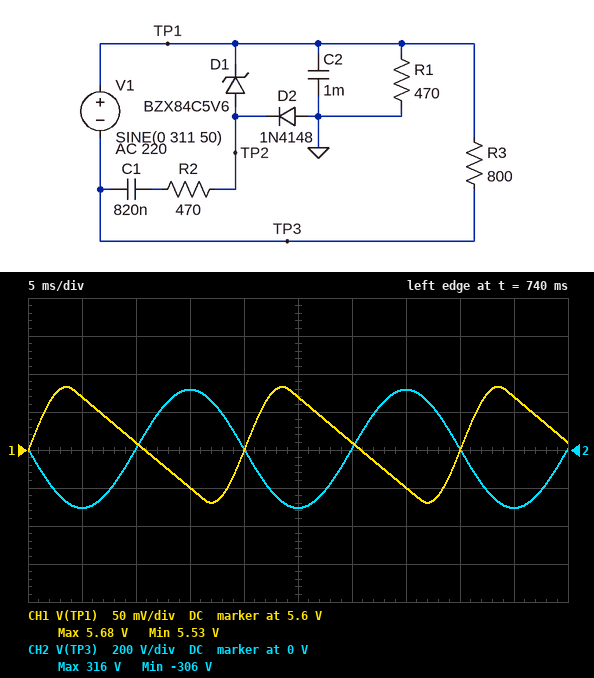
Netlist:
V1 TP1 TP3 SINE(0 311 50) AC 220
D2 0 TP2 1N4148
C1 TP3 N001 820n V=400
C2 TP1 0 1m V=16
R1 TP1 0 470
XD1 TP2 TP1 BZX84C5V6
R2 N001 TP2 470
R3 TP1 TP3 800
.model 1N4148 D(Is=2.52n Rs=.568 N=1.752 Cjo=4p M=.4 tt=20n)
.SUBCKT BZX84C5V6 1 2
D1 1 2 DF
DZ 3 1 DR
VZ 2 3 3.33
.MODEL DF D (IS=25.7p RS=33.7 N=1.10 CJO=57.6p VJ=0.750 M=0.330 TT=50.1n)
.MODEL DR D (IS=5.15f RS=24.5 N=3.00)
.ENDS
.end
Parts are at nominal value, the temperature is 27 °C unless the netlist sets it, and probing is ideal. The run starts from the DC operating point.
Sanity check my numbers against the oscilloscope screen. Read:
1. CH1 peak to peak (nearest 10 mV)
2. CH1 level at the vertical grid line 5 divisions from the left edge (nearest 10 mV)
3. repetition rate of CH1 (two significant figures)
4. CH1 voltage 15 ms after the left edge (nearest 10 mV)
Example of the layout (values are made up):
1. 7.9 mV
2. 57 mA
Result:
1. 150 mV
2. 5.67 V
3. 50 Hz
4. 5.55 V
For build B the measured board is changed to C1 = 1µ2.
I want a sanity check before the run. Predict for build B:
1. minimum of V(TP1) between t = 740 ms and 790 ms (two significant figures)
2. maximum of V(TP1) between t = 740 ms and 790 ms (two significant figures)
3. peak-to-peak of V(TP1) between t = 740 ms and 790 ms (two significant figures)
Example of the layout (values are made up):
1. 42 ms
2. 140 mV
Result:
1. 6.2 V
2. 6.3 V
3. 180 mV
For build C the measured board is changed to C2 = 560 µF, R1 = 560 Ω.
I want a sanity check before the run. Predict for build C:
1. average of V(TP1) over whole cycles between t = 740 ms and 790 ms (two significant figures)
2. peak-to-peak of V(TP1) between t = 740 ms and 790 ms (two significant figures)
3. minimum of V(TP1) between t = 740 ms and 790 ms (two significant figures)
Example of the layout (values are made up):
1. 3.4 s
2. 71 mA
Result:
1. 5.7 V
2. 240 mV
3. 5.6 V
